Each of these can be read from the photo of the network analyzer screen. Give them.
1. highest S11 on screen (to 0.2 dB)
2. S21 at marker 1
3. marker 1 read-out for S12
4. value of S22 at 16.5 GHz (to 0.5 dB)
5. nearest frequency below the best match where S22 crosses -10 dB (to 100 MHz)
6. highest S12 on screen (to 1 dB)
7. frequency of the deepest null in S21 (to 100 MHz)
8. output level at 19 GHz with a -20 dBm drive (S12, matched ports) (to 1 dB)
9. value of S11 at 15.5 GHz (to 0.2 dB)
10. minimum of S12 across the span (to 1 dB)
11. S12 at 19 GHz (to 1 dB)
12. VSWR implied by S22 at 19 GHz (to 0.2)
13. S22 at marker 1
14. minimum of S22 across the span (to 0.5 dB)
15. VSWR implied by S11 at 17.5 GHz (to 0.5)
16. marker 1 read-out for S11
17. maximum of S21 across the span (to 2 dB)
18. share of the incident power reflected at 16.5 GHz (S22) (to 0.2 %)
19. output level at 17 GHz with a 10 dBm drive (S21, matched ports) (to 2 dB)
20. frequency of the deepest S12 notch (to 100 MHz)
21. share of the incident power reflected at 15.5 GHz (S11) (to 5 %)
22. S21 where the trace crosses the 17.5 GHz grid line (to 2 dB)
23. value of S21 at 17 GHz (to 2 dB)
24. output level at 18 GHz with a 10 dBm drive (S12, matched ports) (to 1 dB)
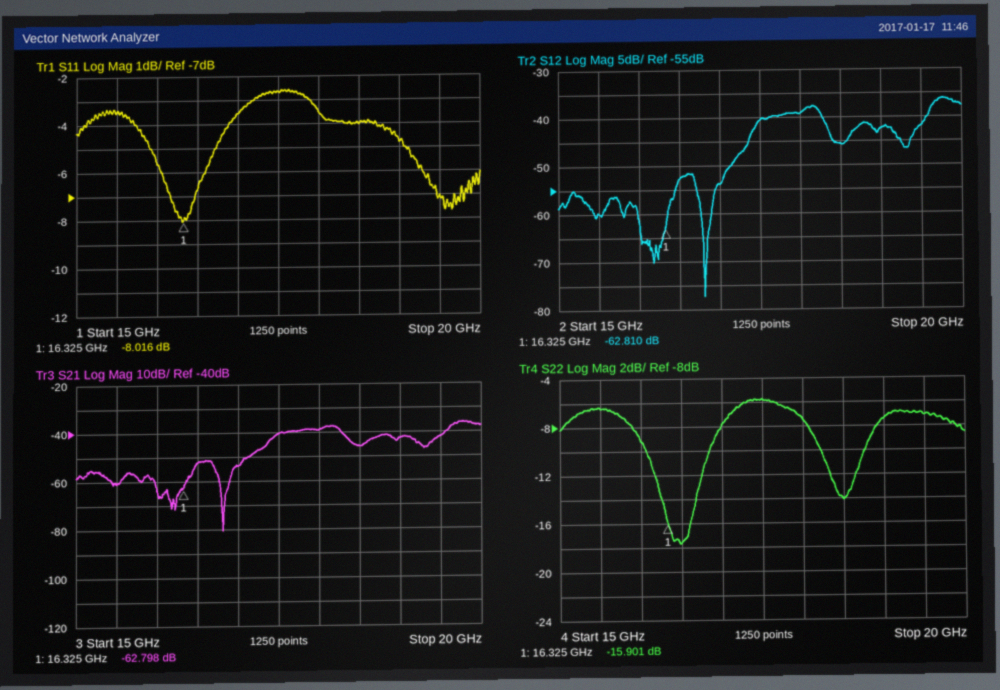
-2.6 dB
-62.798 dB
-62.810 dB
-17.5 dB
16.1 GHz
-36 dB
16.8 GHz
-62 dBm
-3.4 dB
-77 dB
-42 dB
2.4
-15.901 dB
-17.5 dB
6.5
-8.016 dB
-36 dB
1.8 %
-44 dBm
16.8 GHz
45 %
-40 dB
-54 dB
-29 dBm
